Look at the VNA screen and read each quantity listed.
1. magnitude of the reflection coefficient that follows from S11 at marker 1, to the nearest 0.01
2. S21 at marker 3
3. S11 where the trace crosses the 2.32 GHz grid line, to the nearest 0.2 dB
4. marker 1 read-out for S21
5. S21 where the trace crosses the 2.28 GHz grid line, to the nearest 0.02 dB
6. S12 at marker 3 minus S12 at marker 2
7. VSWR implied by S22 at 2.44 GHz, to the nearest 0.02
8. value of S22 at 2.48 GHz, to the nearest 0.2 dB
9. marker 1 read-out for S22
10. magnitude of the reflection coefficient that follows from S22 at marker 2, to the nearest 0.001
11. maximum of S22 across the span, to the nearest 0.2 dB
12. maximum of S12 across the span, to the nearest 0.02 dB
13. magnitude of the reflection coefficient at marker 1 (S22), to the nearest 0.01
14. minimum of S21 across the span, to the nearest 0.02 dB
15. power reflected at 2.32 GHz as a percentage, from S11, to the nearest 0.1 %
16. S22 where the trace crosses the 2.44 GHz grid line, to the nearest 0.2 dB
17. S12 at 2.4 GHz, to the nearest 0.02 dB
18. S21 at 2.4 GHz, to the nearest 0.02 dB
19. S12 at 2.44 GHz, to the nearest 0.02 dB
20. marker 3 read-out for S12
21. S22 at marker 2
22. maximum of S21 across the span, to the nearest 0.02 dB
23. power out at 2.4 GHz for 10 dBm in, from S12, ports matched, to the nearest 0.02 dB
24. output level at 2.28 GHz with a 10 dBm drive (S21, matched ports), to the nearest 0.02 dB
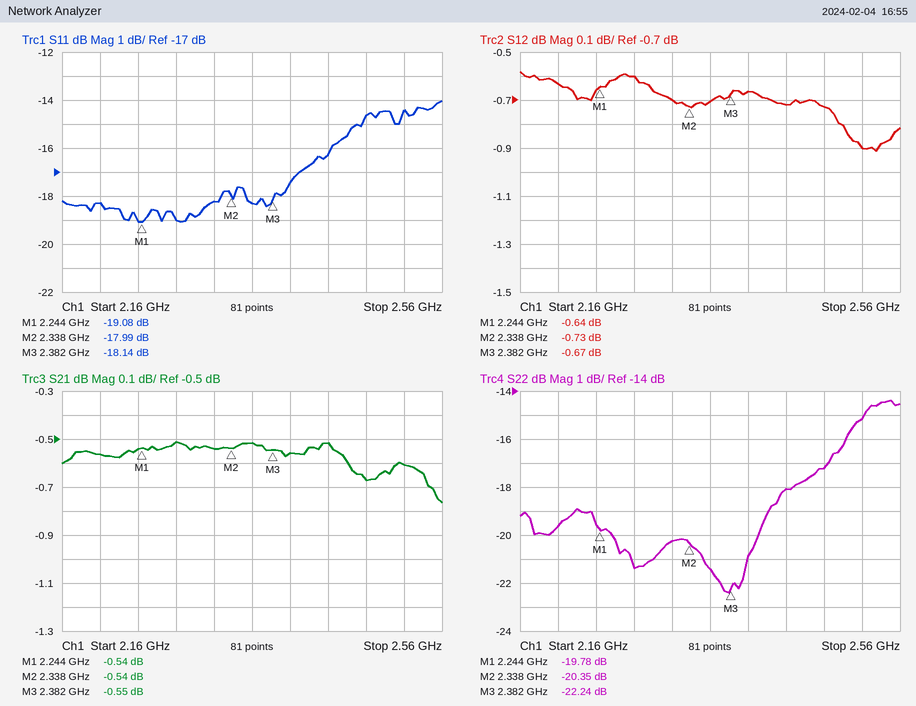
0.11
-0.55 dB
-18.2 dB
-0.54 dB
-0.52 dB
0.06 dB
1.28
-17.2 dB
-19.78 dB
0.096
-14.4 dB
-0.58 dB
0.10
-0.76 dB
1.5 %
-18.0 dB
-0.66 dB
-0.56 dB
-0.72 dB
-0.67 dB
-20.35 dB
-0.52 dB
9.34 dBm
9.48 dBm
